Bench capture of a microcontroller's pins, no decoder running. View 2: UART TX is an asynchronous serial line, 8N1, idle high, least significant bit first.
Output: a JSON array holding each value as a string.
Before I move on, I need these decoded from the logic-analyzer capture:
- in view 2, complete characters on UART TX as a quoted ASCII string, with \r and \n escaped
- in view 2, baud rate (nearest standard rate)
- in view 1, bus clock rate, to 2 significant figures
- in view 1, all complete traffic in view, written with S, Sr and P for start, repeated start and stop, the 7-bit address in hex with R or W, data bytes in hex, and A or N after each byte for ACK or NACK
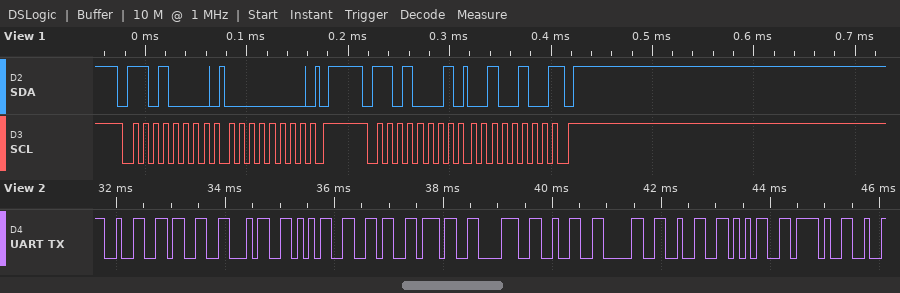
["\"23456782025/\"", "9600 baud", "100 kHz", "S 68W A 00 A P S 68R A 24 N P"]
